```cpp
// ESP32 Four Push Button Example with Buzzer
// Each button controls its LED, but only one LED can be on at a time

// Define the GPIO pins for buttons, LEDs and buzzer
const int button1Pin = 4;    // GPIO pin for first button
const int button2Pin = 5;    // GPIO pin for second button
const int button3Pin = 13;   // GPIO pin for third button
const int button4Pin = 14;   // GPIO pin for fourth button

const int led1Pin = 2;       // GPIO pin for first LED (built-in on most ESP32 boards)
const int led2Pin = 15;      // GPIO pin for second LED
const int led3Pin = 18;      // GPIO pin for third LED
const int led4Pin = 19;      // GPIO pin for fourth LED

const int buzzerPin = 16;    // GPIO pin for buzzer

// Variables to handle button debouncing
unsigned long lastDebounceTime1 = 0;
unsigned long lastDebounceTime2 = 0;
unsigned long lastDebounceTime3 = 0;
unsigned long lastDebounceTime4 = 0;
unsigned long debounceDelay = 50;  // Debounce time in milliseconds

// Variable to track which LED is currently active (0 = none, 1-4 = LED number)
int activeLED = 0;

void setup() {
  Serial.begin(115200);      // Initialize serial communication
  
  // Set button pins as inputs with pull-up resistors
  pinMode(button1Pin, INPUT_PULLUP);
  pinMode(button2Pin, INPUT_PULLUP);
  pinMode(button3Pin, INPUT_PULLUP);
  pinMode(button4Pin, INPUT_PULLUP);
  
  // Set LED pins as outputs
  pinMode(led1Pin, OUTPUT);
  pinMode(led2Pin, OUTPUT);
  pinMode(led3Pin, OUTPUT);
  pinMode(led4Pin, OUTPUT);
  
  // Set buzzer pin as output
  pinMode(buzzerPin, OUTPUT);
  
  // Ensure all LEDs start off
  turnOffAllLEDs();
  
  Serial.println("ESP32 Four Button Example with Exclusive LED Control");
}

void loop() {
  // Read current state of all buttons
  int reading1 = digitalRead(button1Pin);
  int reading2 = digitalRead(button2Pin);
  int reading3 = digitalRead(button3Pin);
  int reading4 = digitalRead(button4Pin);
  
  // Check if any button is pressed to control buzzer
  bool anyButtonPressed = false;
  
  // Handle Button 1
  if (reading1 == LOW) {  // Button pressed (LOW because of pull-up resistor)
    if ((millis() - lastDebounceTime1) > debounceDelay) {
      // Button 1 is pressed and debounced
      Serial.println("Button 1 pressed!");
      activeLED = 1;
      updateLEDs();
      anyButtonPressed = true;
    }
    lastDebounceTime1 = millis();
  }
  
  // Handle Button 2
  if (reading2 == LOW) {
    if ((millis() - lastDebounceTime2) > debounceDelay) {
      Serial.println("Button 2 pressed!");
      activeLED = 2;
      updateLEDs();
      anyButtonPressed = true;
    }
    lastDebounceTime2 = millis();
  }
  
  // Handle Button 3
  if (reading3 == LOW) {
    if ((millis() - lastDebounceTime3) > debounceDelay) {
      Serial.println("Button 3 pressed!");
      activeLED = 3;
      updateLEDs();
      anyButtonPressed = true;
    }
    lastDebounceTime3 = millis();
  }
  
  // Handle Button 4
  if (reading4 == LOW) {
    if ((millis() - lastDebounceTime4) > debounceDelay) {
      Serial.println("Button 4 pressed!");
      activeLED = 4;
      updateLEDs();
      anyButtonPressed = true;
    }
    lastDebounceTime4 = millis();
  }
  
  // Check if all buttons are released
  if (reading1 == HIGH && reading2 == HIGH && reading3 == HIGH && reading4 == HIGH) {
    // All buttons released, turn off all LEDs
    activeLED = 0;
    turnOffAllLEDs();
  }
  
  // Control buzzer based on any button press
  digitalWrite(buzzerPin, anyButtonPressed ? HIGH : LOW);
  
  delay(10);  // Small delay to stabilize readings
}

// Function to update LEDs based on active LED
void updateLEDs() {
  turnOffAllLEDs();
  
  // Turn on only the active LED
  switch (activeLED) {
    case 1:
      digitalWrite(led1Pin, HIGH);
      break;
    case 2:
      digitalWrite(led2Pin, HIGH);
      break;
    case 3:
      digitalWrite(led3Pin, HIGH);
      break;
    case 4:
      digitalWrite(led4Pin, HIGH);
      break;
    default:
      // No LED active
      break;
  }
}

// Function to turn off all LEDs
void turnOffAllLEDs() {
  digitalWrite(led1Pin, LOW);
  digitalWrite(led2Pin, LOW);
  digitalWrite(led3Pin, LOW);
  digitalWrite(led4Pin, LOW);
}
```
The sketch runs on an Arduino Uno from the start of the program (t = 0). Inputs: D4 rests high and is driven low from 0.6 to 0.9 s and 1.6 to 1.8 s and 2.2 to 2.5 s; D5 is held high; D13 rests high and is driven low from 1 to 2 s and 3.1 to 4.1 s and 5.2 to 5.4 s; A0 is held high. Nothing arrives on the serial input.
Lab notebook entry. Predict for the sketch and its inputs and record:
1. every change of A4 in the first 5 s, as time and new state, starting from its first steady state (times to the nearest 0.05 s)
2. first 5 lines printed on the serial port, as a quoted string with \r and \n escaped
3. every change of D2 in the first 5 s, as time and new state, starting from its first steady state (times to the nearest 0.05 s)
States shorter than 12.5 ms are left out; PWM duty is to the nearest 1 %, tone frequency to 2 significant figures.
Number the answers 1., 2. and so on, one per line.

1. 0 s low; 1 s high; 1.6 s low; 3.1 s high; 4.1 s low
2. "ESP32 Four Button Example with Exclusive LED Control\r\nButton 1 pressed!\r\nButton 3 pressed!\r\nButton 1 pressed!\r\nButton 1 pressed!\r\n"
3. 0 s low; 0.6 s high; 0.9 s low; 1.6 s high; 2 s low; 2.2 s high; 2.5 s low
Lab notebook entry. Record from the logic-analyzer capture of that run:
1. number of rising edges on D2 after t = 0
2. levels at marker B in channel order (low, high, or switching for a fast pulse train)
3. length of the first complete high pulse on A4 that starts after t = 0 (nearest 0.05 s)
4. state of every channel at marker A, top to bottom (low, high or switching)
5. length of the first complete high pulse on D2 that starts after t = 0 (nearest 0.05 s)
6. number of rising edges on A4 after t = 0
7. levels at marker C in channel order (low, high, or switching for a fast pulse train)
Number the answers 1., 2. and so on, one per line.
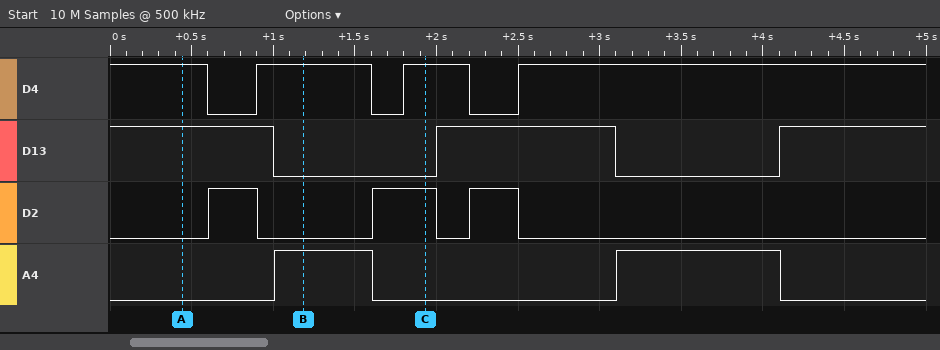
1. 3
2. D4 high, D13 low, D2 low, A4 high
3. 0.60 s
4. D4 high, D13 high, D2 low, A4 low
5. 0.30 s
6. 2
7. D4 high, D13 low, D2 high, A4 low
